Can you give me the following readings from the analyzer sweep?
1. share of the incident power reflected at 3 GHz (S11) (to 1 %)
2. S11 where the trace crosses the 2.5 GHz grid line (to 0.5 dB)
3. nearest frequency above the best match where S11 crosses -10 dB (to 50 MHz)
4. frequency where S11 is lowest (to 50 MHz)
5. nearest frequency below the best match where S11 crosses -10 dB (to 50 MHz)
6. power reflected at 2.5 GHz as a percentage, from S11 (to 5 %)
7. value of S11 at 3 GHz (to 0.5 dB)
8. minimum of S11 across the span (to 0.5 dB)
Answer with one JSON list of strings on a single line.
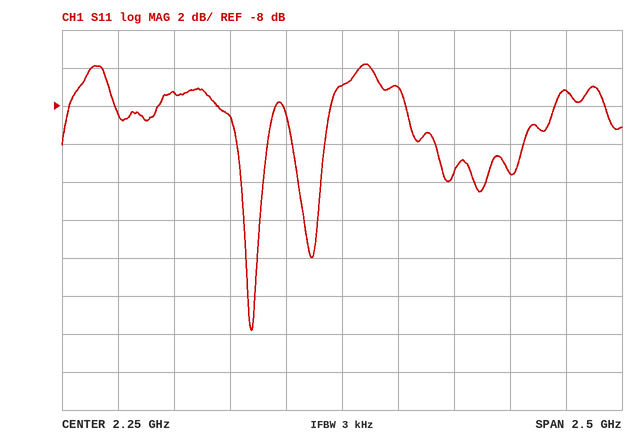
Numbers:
["7 %", "-7.0 dB", "1.90 GHz", "1.85 GHz", "1.80 GHz", "20 %", "-11.5 dB", "-20.0 dB"]
